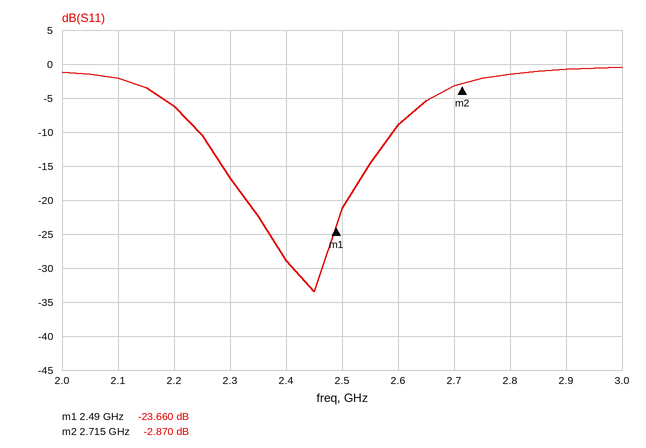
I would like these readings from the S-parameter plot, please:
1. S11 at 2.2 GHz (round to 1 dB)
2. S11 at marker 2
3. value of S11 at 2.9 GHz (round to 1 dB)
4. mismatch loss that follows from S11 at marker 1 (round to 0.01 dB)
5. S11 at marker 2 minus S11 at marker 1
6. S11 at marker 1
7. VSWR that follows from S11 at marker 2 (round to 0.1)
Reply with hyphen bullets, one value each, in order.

- -6 dB
- -2.870 dB
- -1 dB
- 0.02 dB
- 20.790 dB
- -23.660 dB
- 6.1
